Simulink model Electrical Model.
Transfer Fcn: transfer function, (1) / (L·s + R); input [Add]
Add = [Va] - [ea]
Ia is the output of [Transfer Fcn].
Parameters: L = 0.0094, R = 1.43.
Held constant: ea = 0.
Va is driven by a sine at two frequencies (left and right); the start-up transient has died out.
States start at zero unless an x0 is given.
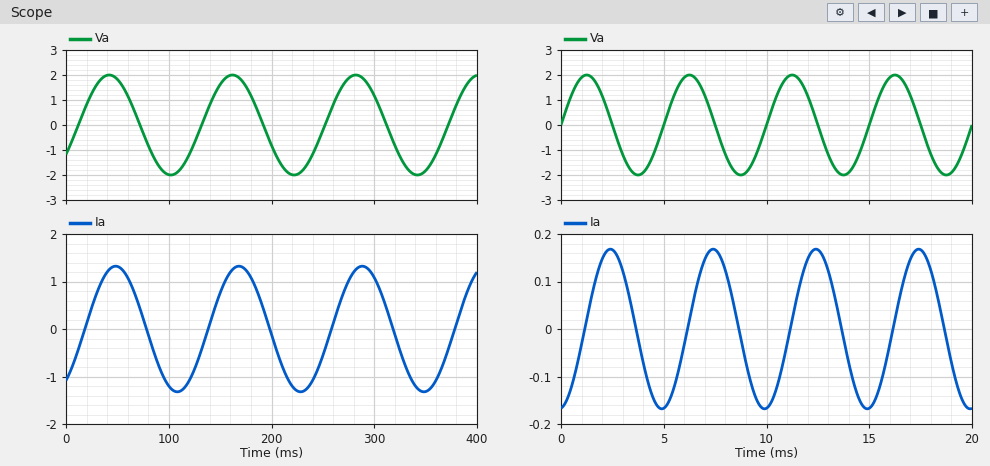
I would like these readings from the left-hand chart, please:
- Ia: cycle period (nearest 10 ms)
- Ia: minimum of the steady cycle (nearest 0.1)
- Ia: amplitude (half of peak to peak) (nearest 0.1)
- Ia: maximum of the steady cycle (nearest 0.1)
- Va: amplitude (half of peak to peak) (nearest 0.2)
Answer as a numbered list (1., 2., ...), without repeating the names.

1. 120 ms
2. -1.3
3. 1.3
4. 1.3
5. 2.0
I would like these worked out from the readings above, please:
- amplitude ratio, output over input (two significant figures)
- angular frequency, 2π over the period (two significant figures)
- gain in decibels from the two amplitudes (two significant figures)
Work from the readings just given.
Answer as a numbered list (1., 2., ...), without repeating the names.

1. 0.65
2. 0.052 rad/ms
3. -3.7 dB
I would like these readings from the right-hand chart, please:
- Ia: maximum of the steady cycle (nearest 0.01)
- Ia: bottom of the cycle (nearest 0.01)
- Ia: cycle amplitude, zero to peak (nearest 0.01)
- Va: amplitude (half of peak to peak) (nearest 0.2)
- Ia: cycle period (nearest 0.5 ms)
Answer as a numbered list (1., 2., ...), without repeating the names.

1. 0.17
2. -0.17
3. 0.17
4. 2.0
5. 5.0 ms
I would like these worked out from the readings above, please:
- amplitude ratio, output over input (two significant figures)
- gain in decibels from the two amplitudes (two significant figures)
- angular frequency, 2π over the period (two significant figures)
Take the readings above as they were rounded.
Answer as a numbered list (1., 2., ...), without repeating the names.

1. 0.085
2. -21 dB
3. 1.3 rad/ms
